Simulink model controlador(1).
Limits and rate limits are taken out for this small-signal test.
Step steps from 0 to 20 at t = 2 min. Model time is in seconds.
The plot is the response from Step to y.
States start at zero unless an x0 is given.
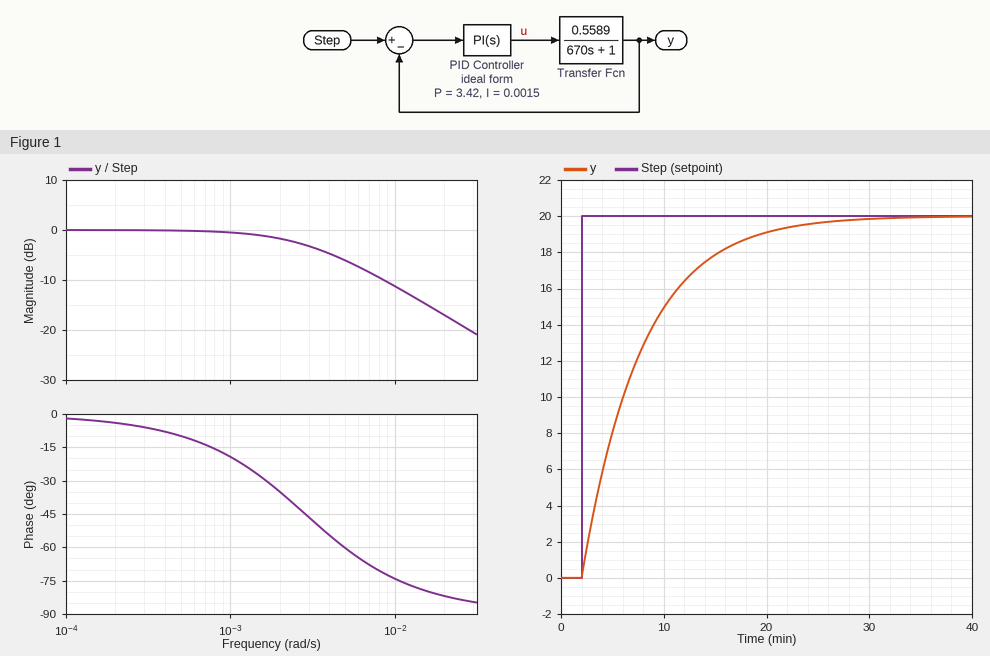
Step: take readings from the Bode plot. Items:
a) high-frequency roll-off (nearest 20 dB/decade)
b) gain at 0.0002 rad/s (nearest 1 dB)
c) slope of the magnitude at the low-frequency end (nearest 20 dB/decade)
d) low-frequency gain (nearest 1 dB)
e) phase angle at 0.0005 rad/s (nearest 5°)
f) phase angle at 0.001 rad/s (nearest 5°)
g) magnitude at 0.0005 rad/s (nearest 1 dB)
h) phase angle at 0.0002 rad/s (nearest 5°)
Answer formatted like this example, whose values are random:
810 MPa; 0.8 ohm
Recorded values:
-20 dB/decade; 0 dB; 0 dB/decade; 0 dB; -10°; -20°; 0 dB; -5°
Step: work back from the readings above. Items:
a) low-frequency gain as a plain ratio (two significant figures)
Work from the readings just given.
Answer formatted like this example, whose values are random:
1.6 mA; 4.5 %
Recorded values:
1.0
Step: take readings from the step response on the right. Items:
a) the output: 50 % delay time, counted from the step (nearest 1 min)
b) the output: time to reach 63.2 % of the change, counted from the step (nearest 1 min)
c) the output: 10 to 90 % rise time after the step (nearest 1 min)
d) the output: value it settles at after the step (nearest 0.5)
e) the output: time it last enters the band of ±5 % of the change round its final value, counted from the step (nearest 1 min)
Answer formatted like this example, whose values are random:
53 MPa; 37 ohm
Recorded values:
4 min; 6 min; 13 min; 20.0; 17 min
